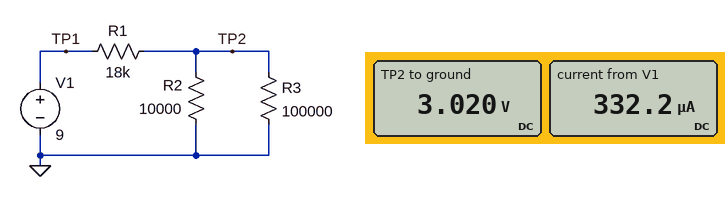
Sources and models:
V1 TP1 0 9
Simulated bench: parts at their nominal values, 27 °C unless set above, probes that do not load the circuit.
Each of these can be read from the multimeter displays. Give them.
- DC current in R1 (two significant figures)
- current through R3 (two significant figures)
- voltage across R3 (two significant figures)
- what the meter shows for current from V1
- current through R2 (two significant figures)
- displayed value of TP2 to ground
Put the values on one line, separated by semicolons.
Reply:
330 µA; 30 µA; 3.0 V; 332.2 µA; 300 µA; 3.020 V
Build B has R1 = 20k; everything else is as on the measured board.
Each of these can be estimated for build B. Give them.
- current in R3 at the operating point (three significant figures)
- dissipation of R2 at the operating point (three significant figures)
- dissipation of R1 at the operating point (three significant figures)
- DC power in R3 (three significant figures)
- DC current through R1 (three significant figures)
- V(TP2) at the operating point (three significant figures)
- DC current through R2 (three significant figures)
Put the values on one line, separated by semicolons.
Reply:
28.1 µA; 791 µW; 1.91 mW; 79.1 µW; 309 µA; 2.81 V; 281 µA
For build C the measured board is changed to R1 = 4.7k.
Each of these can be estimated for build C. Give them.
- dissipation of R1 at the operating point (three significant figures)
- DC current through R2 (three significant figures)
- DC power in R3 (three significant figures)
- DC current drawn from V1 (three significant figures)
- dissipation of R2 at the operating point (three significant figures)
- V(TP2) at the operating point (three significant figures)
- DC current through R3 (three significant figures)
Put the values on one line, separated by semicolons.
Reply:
2.00 mW; 593 µA; 352 µW; 653 µA; 3.52 mW; 5.93 V; 59.3 µA
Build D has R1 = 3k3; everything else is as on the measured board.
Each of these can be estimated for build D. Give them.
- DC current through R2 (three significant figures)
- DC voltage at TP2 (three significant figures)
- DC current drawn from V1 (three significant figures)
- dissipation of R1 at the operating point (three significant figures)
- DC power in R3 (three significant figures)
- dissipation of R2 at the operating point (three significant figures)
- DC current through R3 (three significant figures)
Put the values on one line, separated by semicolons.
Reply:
660 µA; 6.60 V; 726 µA; 1.74 mW; 436 µW; 4.36 mW; 66.0 µA
